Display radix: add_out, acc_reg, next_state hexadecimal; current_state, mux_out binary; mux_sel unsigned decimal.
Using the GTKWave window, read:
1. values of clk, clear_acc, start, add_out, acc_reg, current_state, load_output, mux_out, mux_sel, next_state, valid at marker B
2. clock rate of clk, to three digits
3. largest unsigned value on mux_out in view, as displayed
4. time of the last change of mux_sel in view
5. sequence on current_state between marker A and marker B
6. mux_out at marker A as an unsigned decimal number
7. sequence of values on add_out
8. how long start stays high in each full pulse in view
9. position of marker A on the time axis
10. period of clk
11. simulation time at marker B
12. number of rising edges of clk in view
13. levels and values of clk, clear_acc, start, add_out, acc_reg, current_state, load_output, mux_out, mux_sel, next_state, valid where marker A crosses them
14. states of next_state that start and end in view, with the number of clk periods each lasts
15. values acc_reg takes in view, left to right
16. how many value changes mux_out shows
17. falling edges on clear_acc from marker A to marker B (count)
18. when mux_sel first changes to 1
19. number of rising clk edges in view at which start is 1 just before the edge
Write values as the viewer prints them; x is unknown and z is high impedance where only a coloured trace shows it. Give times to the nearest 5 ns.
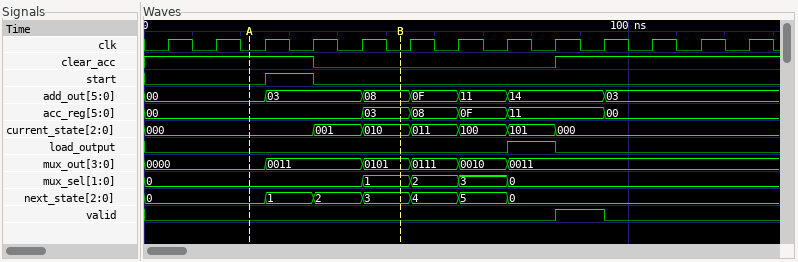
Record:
clk=0, clear_acc=0, start=0, add_out=08, acc_reg=03, current_state=010, load_output=0, mux_out=0101, mux_sel=1, next_state=3, valid=0
100 MHz
0111
75 ns
000, 001, 010
0
00, 03, 08, 0F, 11, 14, 03
10 ns
20 ns
10 ns
55 ns
13
clk=0, clear_acc=1, start=0, add_out=00, acc_reg=00, current_state=000, load_output=0, mux_out=0000, mux_sel=0, next_state=0, valid=0
1: 1, 2: 1, 3: 1, 4: 1, 5: 1
00, 03, 08, 0F, 11, 00
5
1
45 ns
1
